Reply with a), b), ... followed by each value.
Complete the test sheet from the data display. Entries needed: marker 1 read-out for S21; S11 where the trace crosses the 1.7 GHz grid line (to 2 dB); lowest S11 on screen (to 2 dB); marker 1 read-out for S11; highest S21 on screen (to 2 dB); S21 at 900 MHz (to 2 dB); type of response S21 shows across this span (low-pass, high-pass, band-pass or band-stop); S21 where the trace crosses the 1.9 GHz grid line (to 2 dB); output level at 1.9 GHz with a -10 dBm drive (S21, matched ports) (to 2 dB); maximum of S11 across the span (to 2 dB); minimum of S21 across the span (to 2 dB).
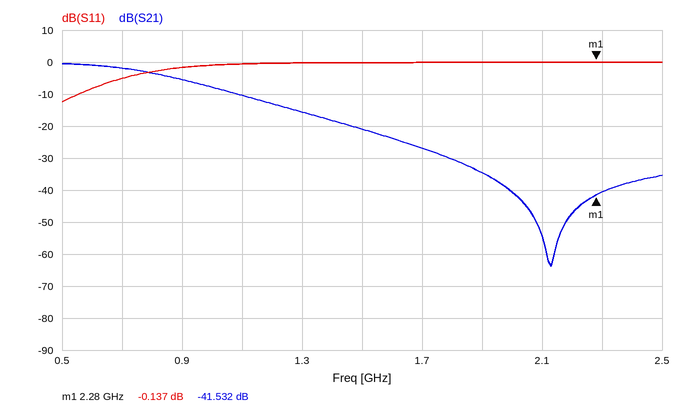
a) -41.532 dB
b) 0 dB
c) -12 dB
d) -0.137 dB
e) 0 dB
f) -6 dB
g) low-pass
h) -34 dB
i) -44 dBm
j) 0 dB
k) -64 dB
